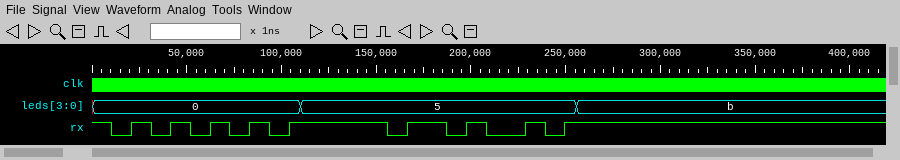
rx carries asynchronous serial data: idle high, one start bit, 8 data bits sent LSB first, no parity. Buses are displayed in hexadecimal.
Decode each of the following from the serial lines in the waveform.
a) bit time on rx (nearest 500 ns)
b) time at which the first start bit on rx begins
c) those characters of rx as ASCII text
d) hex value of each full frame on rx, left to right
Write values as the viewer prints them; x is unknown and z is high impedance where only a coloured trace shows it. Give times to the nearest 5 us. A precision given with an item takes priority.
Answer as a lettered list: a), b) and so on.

a) 10500 ns
b) 10 us
c) "UK"
d) 55, 4B
